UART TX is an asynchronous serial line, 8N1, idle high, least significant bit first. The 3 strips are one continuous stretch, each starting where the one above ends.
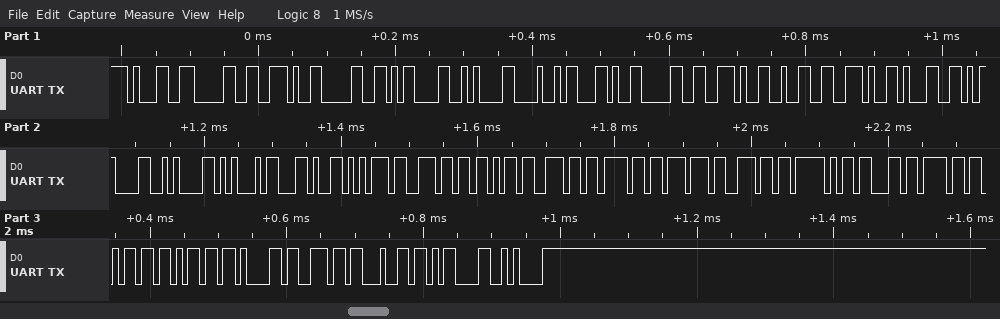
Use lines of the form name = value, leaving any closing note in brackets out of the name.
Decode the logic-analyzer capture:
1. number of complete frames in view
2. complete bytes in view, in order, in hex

number of complete frames in view = 34
complete bytes in view, in order, in hex = 31 30 2E 30 0D 0A 48 2C 30 2E 32 2E 31 0D 0A 45 2C 75 6E 6B 6E 6F 77 6E 5F 63 6F 6D 6D 61 6E 64 0D 0A
